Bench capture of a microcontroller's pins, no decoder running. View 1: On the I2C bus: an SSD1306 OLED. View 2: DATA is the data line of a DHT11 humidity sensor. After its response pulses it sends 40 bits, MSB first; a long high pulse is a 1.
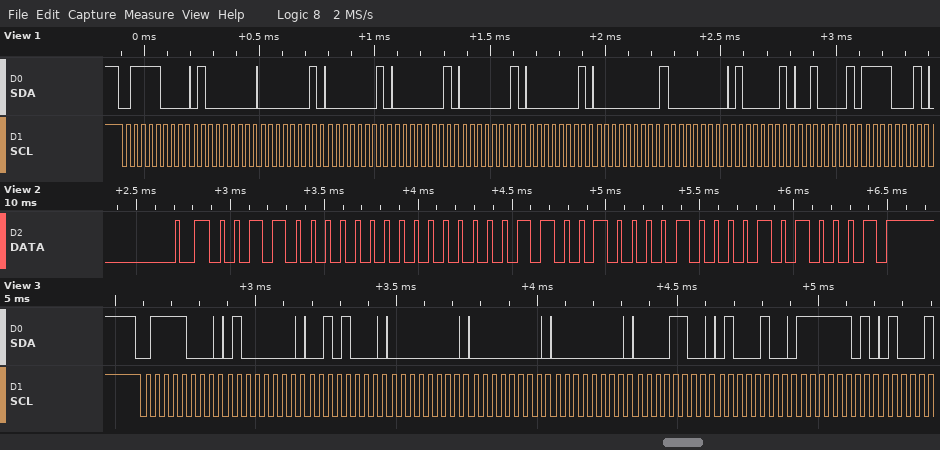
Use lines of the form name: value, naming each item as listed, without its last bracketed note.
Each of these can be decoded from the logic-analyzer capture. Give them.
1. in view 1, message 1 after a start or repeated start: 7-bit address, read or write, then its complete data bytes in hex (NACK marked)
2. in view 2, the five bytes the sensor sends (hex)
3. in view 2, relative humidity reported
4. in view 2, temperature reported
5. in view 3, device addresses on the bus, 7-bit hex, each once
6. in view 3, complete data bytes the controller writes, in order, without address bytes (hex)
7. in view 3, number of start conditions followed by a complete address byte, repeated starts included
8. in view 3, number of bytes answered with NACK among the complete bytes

in view 1, message 1 after a start or repeated start: 7-bit address, read or write, then its complete data bytes in hex: 0x3C write: 40 01 01 01 01 01 00 80 41 21 F1
in view 2, the five bytes the sensor sends: 30 00 19 08 51
in view 2, relative humidity reported: 48 %
in view 2, temperature reported: 25.8 °C
in view 3, device addresses on the bus, 7-bit hex, each once: 0x3C
in view 3, complete data bytes the controller writes, in order, without address bytes: 40 28 00 00 00 0C 44 FD
in view 3, number of start conditions followed by a complete address byte, repeated starts included: 1
in view 3, number of bytes answered with NACK among the complete bytes: 0
